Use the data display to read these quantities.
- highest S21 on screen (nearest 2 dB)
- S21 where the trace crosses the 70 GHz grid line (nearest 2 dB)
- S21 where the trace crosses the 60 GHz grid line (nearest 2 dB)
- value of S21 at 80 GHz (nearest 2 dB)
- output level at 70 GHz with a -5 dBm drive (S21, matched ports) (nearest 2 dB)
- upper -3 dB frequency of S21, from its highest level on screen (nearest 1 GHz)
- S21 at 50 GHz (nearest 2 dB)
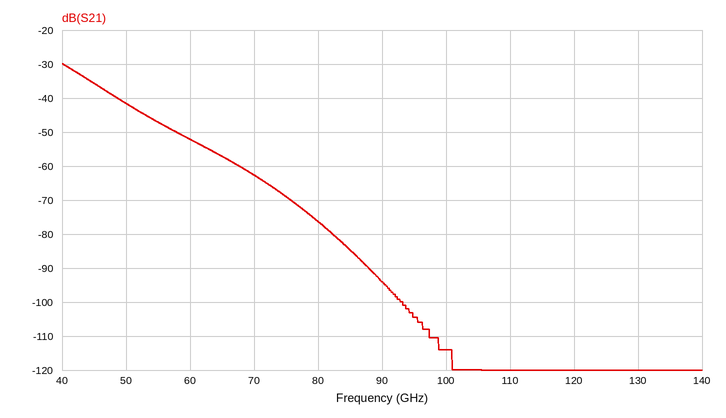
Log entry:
-30 dB
-62 dB
-52 dB
-76 dB
-68 dBm
43 GHz
-42 dB
